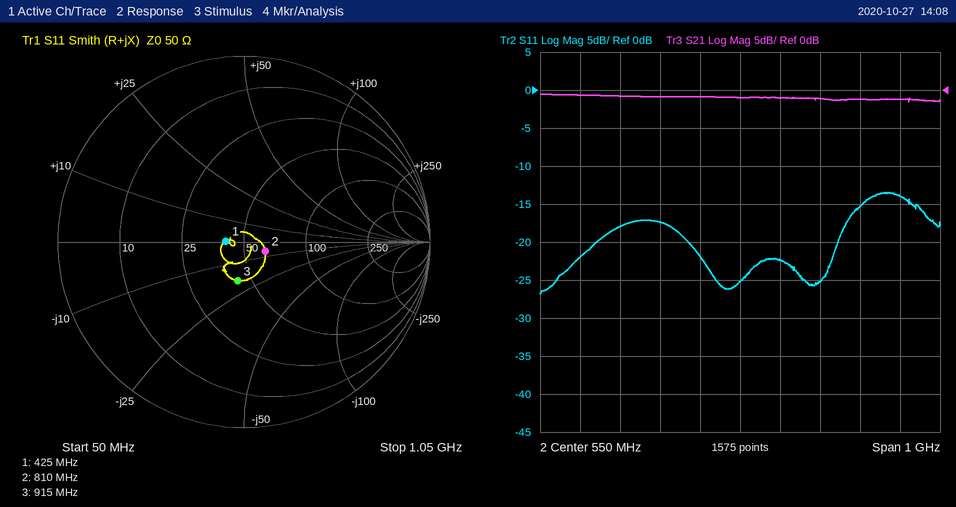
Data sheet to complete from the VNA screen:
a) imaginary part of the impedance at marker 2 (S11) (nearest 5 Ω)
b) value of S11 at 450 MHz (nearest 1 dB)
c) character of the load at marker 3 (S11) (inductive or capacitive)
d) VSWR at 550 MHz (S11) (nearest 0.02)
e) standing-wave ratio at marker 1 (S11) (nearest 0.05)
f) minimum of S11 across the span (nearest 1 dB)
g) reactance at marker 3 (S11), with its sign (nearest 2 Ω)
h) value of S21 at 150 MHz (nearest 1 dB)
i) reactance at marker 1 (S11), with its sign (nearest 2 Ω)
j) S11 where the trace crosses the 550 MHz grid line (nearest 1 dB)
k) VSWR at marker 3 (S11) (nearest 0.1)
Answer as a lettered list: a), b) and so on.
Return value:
a) -5 Ω
b) -22 dB
c) capacitive
d) 1.12
e) 1.20
f) -27 dB
g) -18 Ω
h) -1 dB
i) 0 Ω
j) -25 dB
k) 1.5
